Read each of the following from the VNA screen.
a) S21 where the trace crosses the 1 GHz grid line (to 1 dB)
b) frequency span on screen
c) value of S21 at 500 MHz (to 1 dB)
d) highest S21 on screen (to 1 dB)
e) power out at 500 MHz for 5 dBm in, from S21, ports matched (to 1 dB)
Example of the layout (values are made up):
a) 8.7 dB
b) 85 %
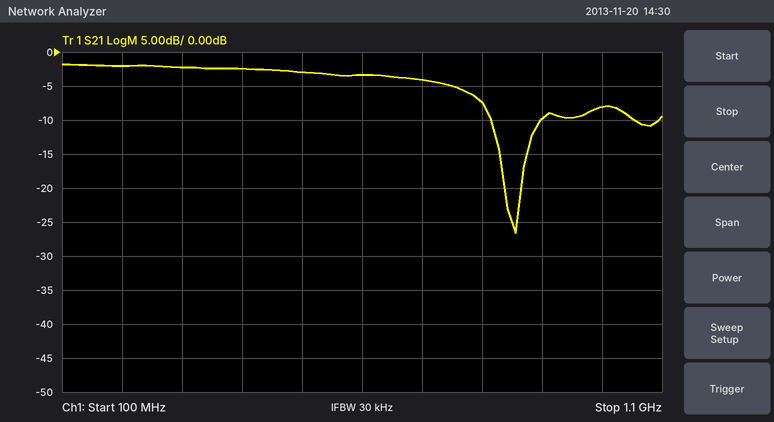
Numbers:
a) -8 dB
b) 1 GHz
c) -3 dB
d) -2 dB
e) 2 dBm
